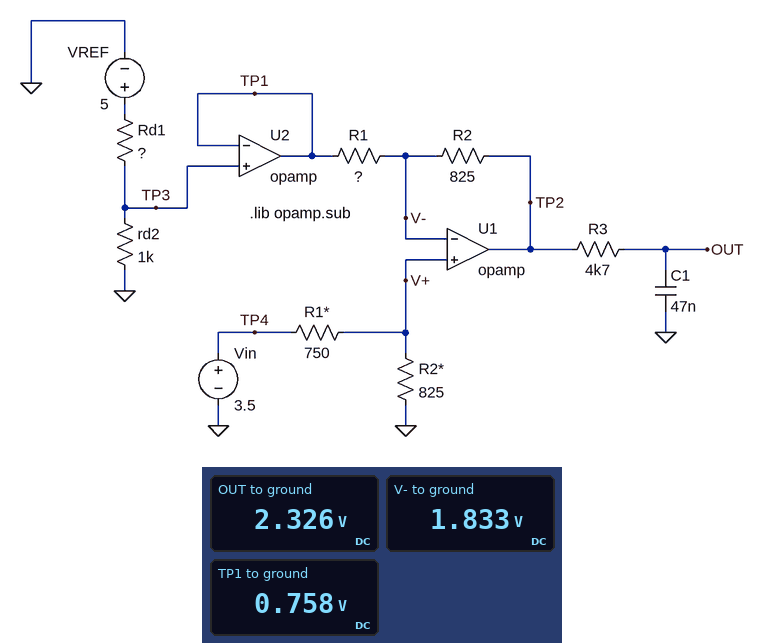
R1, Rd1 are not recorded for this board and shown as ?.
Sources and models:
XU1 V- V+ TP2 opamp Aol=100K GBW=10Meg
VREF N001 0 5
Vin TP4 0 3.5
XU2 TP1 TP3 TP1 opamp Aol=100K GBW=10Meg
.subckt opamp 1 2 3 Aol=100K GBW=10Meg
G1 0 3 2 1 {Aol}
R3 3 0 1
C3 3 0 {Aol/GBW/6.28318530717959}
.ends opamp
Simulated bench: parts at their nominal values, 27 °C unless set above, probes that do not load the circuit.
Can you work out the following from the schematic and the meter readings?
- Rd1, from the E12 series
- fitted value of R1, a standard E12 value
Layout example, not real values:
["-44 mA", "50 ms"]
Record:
["5.6 kΩ", "1.8 kΩ"]
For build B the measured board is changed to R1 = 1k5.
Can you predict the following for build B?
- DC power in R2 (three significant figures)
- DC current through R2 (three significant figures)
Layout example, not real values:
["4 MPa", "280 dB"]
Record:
["424 µW", "717 µA"]
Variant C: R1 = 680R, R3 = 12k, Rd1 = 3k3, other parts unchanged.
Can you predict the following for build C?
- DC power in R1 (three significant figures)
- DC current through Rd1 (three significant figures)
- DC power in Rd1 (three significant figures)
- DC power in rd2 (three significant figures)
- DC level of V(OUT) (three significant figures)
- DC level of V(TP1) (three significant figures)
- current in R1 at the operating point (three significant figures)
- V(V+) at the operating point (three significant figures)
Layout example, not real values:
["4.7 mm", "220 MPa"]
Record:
["661 µW", "1.16 mA", "4.46 mW", "1.35 mW", "2.65 V", "1.16 V", "986 µA", "1.83 V"]
